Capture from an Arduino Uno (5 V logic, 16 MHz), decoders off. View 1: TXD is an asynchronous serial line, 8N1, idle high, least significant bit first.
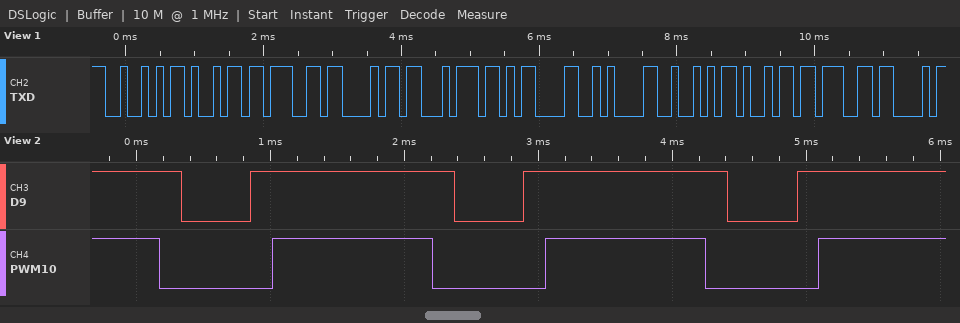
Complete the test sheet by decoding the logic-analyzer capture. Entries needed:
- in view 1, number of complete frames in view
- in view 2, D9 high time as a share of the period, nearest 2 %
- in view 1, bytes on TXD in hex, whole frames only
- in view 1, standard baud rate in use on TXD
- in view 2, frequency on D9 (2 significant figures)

10
74 %
52 69 67 68 74 0D 0A 52 69 67
9600 baud
490 Hz
